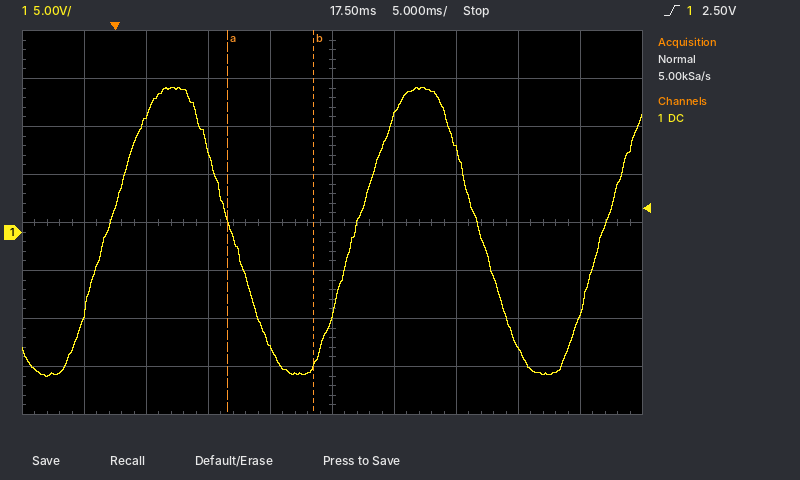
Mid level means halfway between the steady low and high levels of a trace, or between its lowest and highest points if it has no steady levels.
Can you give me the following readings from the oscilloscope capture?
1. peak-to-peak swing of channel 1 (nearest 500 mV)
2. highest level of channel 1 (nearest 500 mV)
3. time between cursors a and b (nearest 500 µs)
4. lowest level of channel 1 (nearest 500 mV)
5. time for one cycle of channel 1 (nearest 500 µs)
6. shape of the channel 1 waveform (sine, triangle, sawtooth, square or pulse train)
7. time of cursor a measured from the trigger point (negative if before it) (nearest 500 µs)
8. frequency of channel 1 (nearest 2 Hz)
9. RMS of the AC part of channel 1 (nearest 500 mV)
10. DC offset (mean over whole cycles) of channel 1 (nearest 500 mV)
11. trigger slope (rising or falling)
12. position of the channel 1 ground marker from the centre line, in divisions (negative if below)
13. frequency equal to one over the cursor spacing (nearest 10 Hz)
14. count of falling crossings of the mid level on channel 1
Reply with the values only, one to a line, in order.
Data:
30.0 V
15.0 V
7.0 ms
-15.0 V
20.0 ms
sine
+9.0 ms
50 Hz
10.5 V
0.0 V
rising
-0.2 div
140 Hz
2
